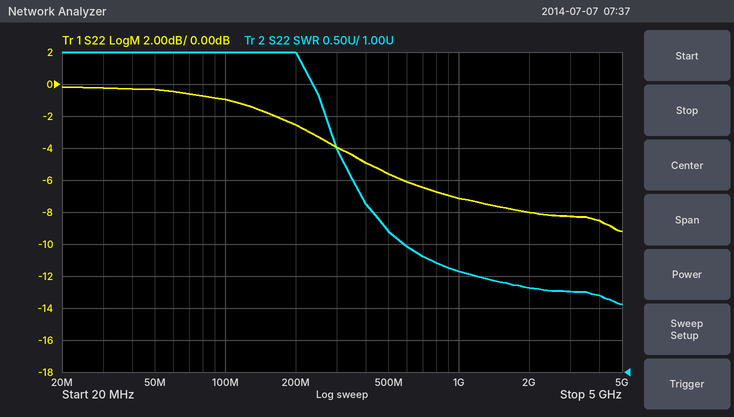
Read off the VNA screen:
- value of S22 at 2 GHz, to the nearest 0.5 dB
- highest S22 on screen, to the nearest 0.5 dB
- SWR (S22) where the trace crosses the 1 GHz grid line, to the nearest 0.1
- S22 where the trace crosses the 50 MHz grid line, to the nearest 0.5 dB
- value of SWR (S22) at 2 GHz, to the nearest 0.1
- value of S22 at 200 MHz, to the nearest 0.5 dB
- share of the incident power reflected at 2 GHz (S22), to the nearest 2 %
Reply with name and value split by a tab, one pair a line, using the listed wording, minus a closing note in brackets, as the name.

value of S22 at 2 GHz, to the nearest 0.5 dB	-8.0 dB
highest S22 on screen, to the nearest 0.5 dB	0.0 dB
SWR (S22) where the trace crosses the 1 GHz grid line, to the nearest 0.1	2.6
S22 where the trace crosses the 50 MHz grid line, to the nearest 0.5 dB	-0.5 dB
value of SWR (S22) at 2 GHz, to the nearest 0.1	2.3
value of S22 at 200 MHz, to the nearest 0.5 dB	-2.5 dB
share of the incident power reflected at 2 GHz (S22), to the nearest 2 %	16 %
